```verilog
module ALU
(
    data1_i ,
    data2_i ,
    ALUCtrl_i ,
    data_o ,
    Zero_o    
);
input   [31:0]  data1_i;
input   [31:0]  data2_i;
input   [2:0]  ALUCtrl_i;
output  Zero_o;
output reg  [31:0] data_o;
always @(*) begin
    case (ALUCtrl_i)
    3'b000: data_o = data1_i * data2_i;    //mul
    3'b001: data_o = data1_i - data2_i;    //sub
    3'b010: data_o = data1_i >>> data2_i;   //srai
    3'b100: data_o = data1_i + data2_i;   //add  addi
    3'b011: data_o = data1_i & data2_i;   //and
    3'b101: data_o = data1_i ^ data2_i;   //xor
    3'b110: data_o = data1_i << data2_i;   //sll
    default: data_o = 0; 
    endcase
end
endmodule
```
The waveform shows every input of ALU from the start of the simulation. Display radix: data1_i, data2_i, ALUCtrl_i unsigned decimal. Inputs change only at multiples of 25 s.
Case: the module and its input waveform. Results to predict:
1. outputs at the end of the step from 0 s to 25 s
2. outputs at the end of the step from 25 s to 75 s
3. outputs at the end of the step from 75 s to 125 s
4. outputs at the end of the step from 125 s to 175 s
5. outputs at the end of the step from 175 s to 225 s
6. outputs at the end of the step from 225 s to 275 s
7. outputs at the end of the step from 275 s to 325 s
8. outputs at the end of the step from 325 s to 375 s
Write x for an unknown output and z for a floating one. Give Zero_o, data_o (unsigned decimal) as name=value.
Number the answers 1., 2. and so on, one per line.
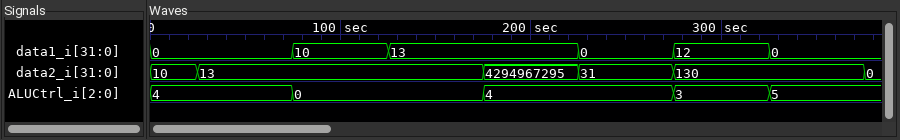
1. Zero_o=z, data_o=10
2. Zero_o=z, data_o=13
3. Zero_o=z, data_o=130
4. Zero_o=z, data_o=169
5. Zero_o=z, data_o=12
6. Zero_o=z, data_o=31
7. Zero_o=z, data_o=0
8. Zero_o=z, data_o=130
